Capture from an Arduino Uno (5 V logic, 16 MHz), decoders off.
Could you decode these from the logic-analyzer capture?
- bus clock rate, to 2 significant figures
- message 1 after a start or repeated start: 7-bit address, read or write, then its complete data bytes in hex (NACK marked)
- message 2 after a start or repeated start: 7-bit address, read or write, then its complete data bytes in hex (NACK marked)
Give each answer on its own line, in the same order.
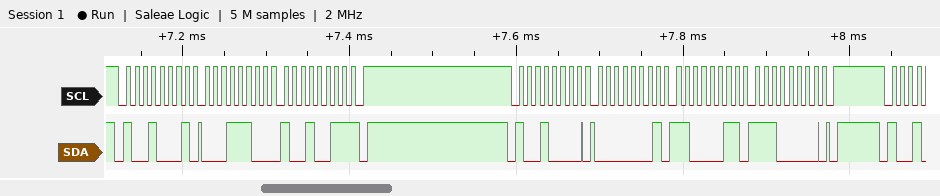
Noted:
100 kHz
0x48 read: 1C 93 NACK
0x48 write: 01 C3 E0
